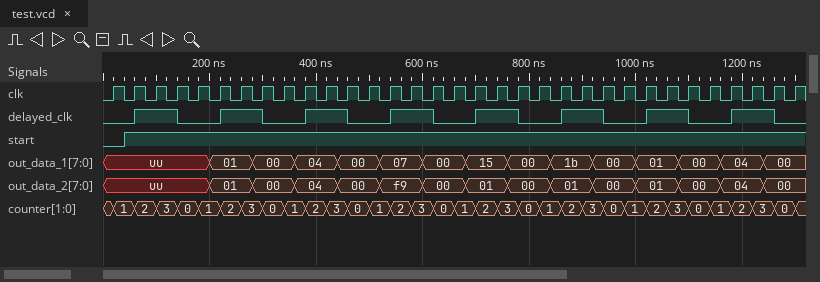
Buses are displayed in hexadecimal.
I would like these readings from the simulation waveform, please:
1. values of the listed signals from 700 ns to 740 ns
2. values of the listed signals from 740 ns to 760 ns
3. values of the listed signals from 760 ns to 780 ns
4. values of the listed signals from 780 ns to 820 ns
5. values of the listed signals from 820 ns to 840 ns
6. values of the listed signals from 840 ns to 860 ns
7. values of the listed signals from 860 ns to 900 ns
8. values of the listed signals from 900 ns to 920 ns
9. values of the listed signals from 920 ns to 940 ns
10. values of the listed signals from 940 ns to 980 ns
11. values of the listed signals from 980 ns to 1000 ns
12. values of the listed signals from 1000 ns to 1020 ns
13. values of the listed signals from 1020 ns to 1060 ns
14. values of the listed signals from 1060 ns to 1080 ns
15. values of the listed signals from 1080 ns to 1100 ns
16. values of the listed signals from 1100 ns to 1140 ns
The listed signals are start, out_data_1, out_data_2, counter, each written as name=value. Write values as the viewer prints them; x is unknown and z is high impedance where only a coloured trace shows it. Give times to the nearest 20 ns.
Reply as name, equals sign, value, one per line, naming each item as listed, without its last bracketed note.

values of the listed signals from 700 ns to 740 ns = start=1, out_data_1=15, out_data_2=01, counter=2
values of the listed signals from 740 ns to 760 ns = start=1, out_data_1=15, out_data_2=01, counter=3
values of the listed signals from 760 ns to 780 ns = start=1, out_data_1=00, out_data_2=00, counter=3
values of the listed signals from 780 ns to 820 ns = start=1, out_data_1=00, out_data_2=00, counter=0
values of the listed signals from 820 ns to 840 ns = start=1, out_data_1=00, out_data_2=00, counter=1
values of the listed signals from 840 ns to 860 ns = start=1, out_data_1=1b, out_data_2=01, counter=1
values of the listed signals from 860 ns to 900 ns = start=1, out_data_1=1b, out_data_2=01, counter=2
values of the listed signals from 900 ns to 920 ns = start=1, out_data_1=1b, out_data_2=01, counter=3
values of the listed signals from 920 ns to 940 ns = start=1, out_data_1=00, out_data_2=00, counter=3
values of the listed signals from 940 ns to 980 ns = start=1, out_data_1=00, out_data_2=00, counter=0
values of the listed signals from 980 ns to 1000 ns = start=1, out_data_1=00, out_data_2=00, counter=1
values of the listed signals from 1000 ns to 1020 ns = start=1, out_data_1=01, out_data_2=01, counter=1
values of the listed signals from 1020 ns to 1060 ns = start=1, out_data_1=01, out_data_2=01, counter=2
values of the listed signals from 1060 ns to 1080 ns = start=1, out_data_1=01, out_data_2=01, counter=3
values of the listed signals from 1080 ns to 1100 ns = start=1, out_data_1=00, out_data_2=00, counter=3
values of the listed signals from 1100 ns to 1140 ns = start=1, out_data_1=00, out_data_2=00, counter=0
